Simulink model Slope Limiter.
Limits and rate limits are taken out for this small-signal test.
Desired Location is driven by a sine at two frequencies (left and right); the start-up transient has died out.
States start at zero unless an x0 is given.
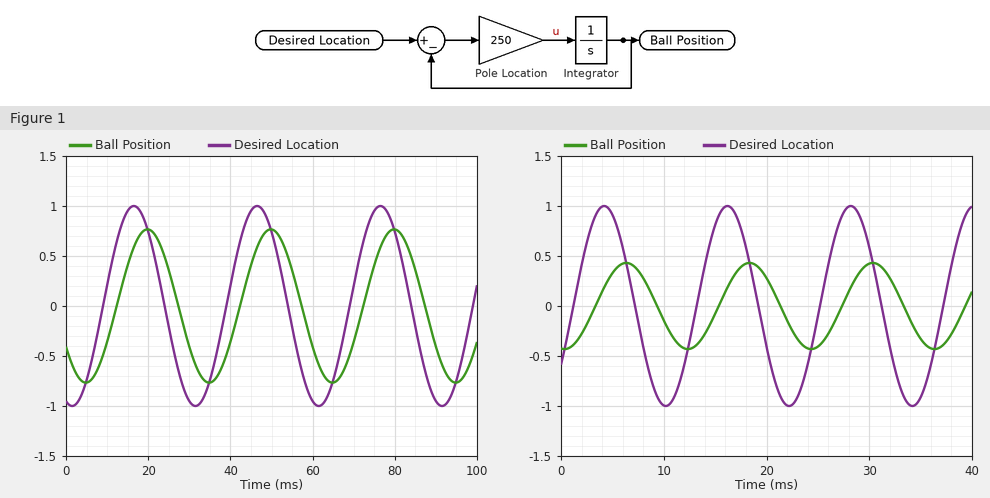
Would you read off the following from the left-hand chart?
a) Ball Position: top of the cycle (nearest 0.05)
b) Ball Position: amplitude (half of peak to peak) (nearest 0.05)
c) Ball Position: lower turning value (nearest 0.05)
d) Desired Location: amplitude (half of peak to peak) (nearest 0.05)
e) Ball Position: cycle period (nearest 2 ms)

0.75
0.75
-0.75
1.00
30 ms
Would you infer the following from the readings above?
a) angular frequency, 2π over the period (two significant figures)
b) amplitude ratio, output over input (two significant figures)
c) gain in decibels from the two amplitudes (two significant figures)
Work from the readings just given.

0.21 rad/ms
0.75
-2.5 dB
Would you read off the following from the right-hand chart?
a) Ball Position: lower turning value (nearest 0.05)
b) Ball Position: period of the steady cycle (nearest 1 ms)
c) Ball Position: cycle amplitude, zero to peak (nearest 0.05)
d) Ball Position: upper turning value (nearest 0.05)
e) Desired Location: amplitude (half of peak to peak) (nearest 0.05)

-0.45
12 ms
0.45
0.45
1.00
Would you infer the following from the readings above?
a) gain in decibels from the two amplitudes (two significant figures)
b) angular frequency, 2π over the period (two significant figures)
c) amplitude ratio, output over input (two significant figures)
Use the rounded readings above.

-6.9 dB
0.52 rad/ms
0.45
